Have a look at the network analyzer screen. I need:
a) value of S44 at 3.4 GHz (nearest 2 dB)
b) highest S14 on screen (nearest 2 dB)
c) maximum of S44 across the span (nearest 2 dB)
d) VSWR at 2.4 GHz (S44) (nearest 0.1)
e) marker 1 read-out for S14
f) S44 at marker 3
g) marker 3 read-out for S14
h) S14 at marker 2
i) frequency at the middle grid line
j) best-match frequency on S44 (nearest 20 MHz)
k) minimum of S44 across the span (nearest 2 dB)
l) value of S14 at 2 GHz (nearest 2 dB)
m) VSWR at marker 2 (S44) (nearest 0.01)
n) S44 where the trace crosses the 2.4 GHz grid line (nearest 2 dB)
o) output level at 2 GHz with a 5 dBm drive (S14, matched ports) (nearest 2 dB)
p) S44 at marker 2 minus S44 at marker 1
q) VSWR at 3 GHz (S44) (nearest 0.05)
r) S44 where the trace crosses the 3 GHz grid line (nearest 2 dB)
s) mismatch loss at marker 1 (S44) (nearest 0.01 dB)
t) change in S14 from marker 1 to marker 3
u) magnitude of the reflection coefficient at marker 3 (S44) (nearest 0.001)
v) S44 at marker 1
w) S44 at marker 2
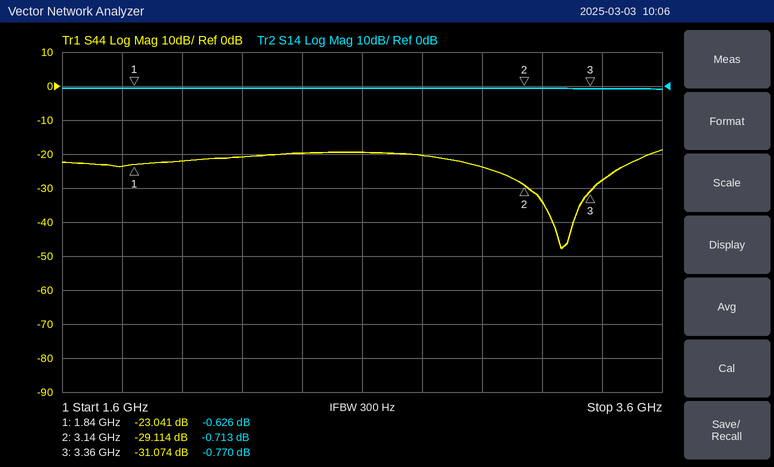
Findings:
-28 dB
0 dB
-18 dB
1.2
-0.626 dB
-31.074 dB
-0.770 dB
-0.713 dB
2.6 GHz
3.26 GHz
-48 dB
0 dB
1.07
-20 dB
4 dBm
-6.073 dB
1.15
-24 dB
0.02 dB
-0.144 dB
0.028
-23.041 dB
-29.114 dB
